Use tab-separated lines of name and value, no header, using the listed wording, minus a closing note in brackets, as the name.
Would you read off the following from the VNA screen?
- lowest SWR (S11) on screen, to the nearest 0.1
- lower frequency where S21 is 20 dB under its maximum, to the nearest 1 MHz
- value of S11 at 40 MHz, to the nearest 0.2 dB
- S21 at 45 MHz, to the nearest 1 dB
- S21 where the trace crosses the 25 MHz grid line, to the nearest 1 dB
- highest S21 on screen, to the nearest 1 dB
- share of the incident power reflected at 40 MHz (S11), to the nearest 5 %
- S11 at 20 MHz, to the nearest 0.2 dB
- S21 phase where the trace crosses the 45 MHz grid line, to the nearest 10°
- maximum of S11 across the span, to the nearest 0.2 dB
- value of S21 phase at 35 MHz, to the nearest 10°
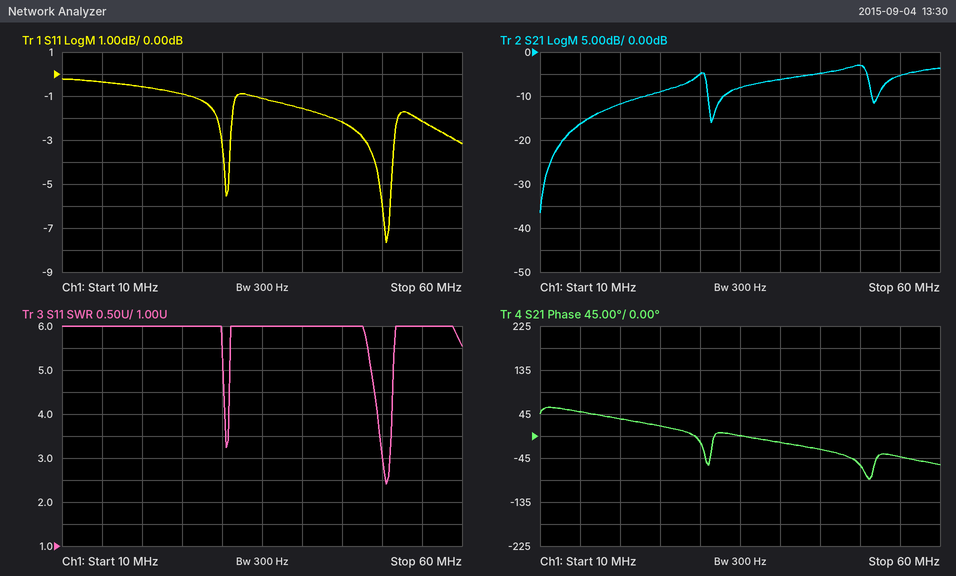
lowest SWR (S11) on screen, to the nearest 0.1	2.4
lower frequency where S21 is 20 dB under its maximum, to the nearest 1 MHz	12 MHz
value of S11 at 40 MHz, to the nearest 0.2 dB	-1.6 dB
S21 at 45 MHz, to the nearest 1 dB	-5 dB
S21 where the trace crosses the 25 MHz grid line, to the nearest 1 dB	-9 dB
highest S21 on screen, to the nearest 1 dB	-3 dB
share of the incident power reflected at 40 MHz (S11), to the nearest 5 %	70 %
S11 at 20 MHz, to the nearest 0.2 dB	-0.6 dB
S21 phase where the trace crosses the 45 MHz grid line, to the nearest 10°	-30°
maximum of S11 across the span, to the nearest 0.2 dB	-0.2 dB
value of S21 phase at 35 MHz, to the nearest 10°	0°
